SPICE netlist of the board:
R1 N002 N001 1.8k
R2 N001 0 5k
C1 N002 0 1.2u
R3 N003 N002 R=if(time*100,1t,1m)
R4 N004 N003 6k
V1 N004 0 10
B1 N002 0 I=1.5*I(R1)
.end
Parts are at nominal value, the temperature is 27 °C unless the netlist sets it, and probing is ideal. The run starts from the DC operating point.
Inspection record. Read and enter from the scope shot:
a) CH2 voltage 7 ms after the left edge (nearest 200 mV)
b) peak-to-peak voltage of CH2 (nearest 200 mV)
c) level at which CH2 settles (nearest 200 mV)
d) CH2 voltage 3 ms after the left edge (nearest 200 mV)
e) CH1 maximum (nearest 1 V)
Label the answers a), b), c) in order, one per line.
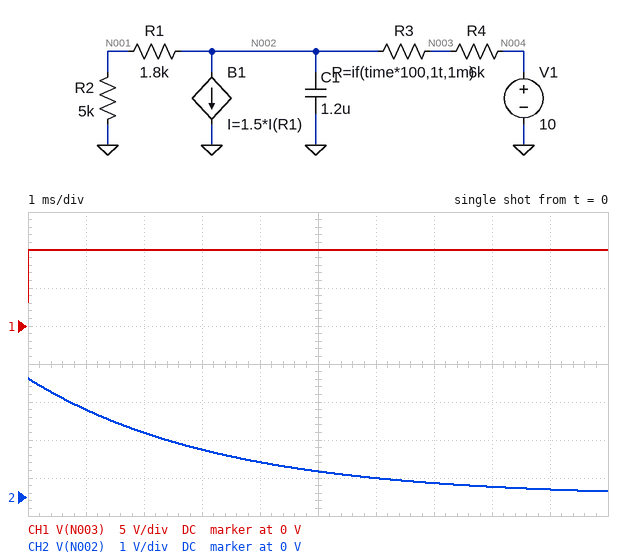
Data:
a) 400 mV
b) 3.0 V
c) 200 mV
d) 1.2 V
e) 10 V
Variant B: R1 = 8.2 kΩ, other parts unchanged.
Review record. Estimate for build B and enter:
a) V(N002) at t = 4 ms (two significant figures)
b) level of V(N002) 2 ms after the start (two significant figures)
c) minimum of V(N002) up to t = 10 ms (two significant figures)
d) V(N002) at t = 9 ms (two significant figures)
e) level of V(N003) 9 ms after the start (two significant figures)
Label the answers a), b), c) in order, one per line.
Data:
a) 2.5 V
b) 3.4 V
c) 970 mV
d) 1.1 V
e) 10 V
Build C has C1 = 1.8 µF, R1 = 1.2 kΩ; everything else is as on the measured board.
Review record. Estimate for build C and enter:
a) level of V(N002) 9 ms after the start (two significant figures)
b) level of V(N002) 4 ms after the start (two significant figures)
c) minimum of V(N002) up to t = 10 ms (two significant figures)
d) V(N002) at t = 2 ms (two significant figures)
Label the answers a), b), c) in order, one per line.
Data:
a) 390 mV
b) 1.2 V
c) 310 mV
d) 1.9 V
